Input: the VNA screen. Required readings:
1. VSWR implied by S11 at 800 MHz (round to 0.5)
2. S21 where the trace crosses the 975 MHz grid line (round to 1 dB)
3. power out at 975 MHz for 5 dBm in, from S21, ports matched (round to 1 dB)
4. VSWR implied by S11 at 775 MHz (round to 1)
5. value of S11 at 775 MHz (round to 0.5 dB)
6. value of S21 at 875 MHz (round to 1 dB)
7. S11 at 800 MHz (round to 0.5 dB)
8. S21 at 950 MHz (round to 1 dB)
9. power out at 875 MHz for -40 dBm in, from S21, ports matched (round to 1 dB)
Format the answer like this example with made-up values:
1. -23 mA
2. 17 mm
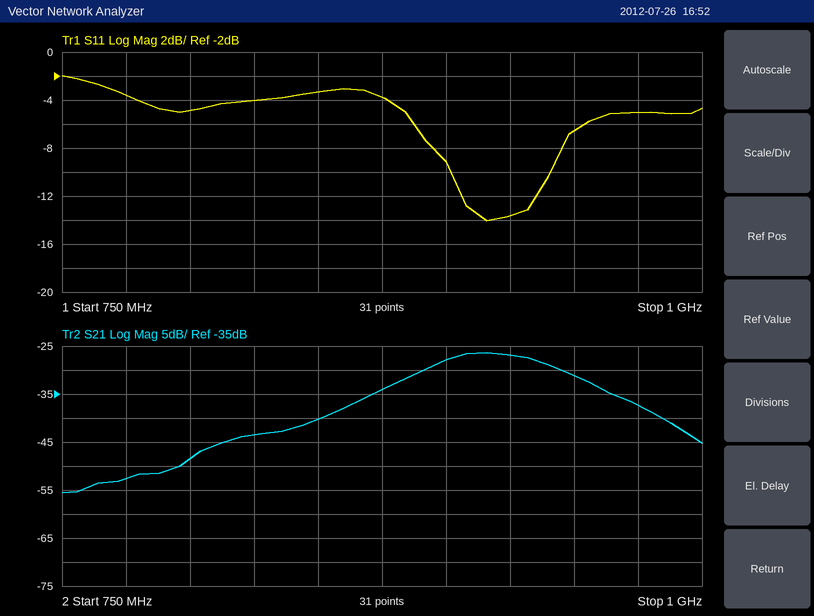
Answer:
1. 3.5
2. -37 dB
3. -32 dBm
4. 5
5. -3.5 dB
6. -34 dB
7. -5.0 dB
8. -31 dB
9. -74 dBm
